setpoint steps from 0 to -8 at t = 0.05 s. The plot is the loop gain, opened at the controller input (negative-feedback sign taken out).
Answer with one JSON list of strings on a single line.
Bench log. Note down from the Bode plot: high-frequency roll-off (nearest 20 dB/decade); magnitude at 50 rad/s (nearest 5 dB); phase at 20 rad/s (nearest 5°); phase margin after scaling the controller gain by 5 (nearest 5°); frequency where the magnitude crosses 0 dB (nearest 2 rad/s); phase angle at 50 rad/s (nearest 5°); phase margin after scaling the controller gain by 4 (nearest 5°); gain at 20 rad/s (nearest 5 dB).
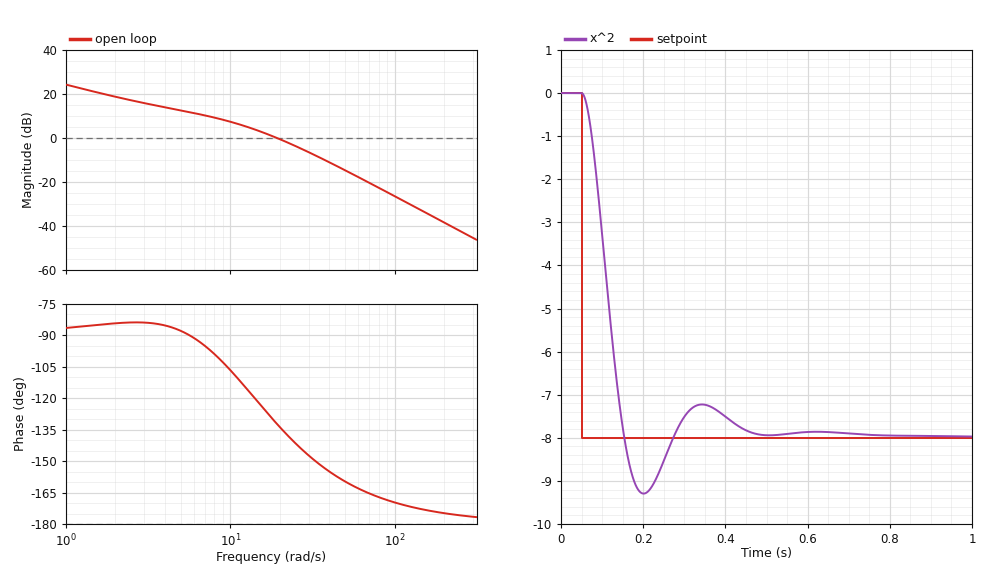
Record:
["-40 dB/decade", "-15 dB", "-135°", "20°", "20 rad/s", "-160°", "25°", "0 dB"]
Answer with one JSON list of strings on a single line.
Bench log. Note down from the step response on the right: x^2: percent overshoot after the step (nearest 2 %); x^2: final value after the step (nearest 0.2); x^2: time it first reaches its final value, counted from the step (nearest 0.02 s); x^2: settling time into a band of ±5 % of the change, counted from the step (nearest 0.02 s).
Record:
["16 %", "-8.0", "0.10 s", "0.36 s"]
